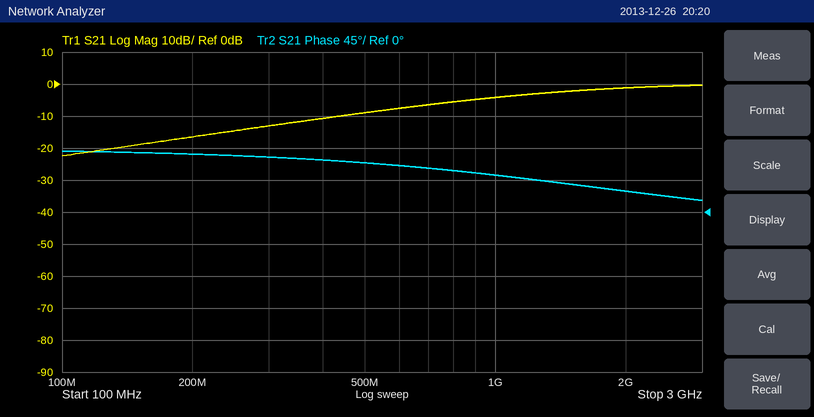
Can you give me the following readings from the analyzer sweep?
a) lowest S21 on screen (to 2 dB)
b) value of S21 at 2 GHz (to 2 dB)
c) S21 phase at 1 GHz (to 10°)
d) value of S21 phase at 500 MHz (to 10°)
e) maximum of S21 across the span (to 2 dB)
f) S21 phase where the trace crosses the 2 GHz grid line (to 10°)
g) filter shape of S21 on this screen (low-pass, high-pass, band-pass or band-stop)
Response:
-22 dB
-2 dB
50°
70°
0 dB
30°
high-pass
